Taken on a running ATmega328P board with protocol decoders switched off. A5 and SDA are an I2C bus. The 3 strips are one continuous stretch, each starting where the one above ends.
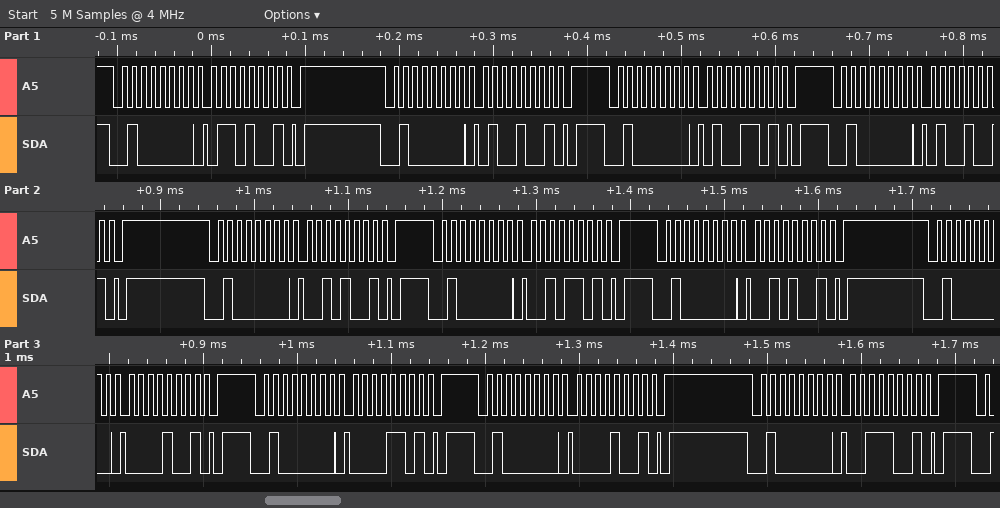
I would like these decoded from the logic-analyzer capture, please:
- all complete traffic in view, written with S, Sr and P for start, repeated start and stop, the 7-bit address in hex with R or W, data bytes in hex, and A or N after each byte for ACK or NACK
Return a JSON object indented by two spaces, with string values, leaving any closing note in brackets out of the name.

{
  "all complete traffic in view, written with S, Sr and P for start, repeated start and stop, the 7-bit address in hex with R or W, data bytes in hex, and A or N after each byte for ACK or NACK": "S 20W A 69 A P S 20W A 49 A P S 20W A 4D A P S 20W A 49 A P S 20W A 29 A P S 20W A 2D A P S 20W A 29 A P S 20W A 09 A P S 20W A 0D A P S 20W A 09 A P S 20W A 39 A P"
}
